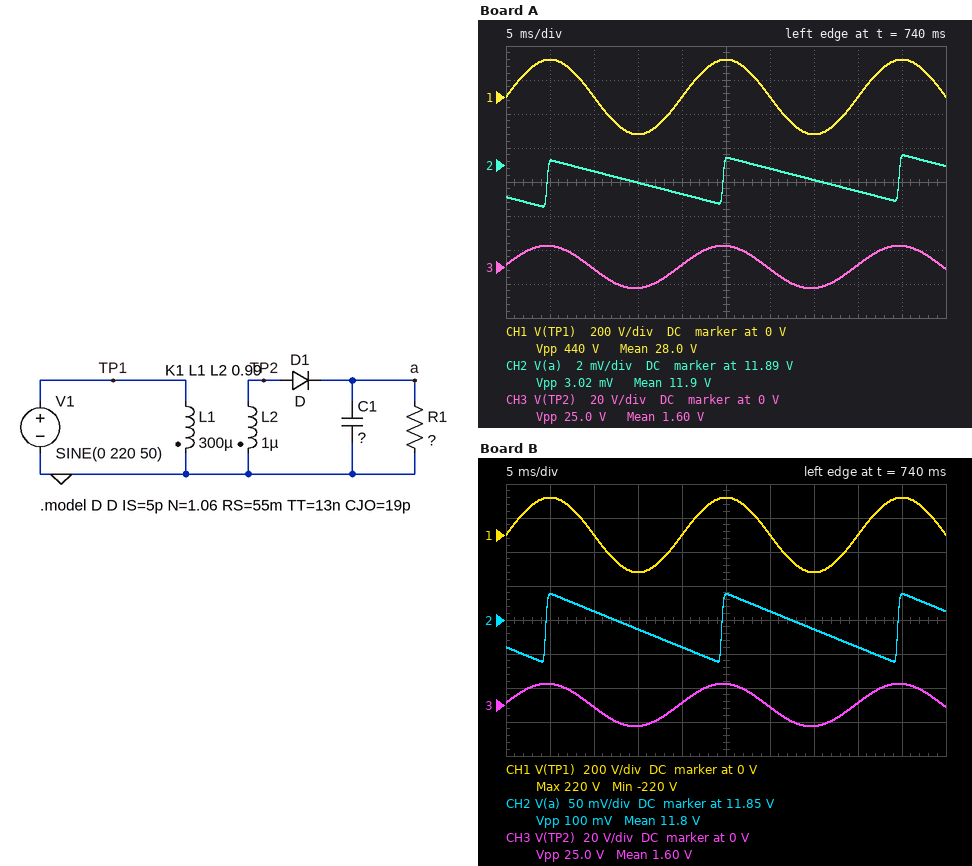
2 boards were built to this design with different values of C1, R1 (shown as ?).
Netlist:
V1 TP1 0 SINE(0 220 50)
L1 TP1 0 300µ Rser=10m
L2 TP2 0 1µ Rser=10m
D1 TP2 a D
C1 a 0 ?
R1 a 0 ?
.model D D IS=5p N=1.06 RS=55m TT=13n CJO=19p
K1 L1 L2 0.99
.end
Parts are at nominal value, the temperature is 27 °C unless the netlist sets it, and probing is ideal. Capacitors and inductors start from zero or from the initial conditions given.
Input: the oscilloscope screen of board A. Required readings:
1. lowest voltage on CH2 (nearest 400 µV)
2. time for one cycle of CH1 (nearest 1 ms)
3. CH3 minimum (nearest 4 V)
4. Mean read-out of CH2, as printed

11.8896 V
20 ms
-12 V
11.9 V
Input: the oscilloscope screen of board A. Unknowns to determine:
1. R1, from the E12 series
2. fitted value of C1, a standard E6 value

27 kΩ
3.3 mF
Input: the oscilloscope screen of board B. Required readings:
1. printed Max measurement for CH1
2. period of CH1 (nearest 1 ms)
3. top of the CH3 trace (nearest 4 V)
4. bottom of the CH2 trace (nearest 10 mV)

220 V
20 ms
12 V
11.79 V
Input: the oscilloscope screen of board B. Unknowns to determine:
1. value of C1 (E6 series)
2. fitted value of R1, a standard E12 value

330 µF
6.8 kΩ
